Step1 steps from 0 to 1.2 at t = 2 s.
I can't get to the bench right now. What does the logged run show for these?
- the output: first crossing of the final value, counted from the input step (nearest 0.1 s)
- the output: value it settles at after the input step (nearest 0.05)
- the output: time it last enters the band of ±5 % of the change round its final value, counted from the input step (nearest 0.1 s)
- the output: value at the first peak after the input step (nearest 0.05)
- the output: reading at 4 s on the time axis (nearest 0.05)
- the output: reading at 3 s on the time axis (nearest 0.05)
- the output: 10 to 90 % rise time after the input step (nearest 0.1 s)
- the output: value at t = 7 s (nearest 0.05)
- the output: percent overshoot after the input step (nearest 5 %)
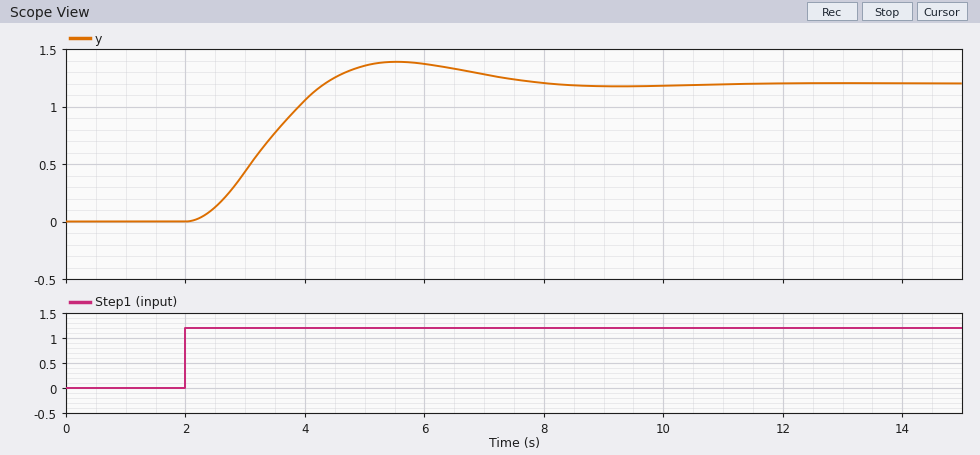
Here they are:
2.3 s
1.20
5.2 s
1.40
1.05
0.45
1.6 s
1.30
15 %
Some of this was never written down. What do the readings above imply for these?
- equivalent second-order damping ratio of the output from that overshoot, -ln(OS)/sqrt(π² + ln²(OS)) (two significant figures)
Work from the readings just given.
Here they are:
0.52
